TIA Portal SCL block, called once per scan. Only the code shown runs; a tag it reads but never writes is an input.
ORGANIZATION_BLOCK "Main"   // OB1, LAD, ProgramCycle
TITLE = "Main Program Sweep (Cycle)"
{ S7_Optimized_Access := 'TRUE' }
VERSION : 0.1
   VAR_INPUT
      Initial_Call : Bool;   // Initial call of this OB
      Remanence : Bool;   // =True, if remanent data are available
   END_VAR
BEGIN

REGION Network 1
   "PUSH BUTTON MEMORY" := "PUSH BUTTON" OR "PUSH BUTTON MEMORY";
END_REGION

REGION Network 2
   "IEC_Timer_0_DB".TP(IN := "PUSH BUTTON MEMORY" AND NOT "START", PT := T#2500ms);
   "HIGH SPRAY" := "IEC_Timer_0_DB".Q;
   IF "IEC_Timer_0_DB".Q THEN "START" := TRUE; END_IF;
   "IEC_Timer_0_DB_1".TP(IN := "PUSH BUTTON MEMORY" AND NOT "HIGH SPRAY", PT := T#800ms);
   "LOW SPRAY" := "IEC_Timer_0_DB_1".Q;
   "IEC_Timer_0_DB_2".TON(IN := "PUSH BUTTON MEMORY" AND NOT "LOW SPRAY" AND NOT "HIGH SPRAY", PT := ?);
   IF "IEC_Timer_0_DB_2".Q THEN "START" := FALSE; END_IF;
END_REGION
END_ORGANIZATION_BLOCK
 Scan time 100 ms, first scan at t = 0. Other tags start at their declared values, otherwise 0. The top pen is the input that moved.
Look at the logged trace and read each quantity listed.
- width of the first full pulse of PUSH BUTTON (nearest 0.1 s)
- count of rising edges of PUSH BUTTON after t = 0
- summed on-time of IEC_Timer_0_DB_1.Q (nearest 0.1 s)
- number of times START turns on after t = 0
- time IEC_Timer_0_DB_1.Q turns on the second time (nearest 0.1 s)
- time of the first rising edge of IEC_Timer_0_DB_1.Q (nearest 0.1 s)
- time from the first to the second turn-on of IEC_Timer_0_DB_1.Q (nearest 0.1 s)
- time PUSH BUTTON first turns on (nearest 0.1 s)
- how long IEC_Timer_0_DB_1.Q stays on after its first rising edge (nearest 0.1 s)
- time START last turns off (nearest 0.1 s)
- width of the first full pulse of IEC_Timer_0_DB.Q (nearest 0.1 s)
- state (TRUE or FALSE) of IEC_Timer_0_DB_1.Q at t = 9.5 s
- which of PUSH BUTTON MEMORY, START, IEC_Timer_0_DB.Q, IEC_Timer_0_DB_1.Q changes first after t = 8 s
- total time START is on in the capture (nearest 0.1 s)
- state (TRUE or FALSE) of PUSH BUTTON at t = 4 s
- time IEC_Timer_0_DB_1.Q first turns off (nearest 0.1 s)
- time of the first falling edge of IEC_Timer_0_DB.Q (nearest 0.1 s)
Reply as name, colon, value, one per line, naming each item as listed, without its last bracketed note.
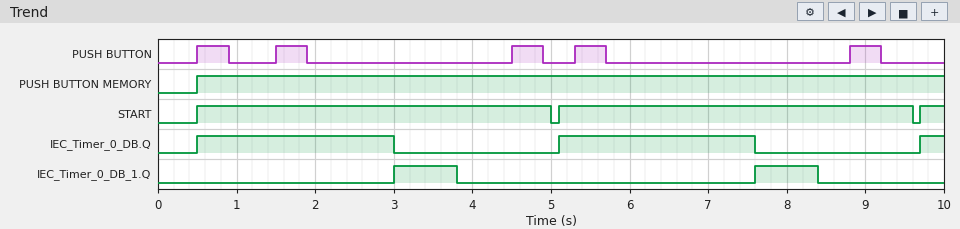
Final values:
width of the first full pulse of PUSH BUTTON: 0.4 s
count of rising edges of PUSH BUTTON after t = 0: 5
summed on-time of IEC_Timer_0_DB_1.Q: 1.6 s
number of times START turns on after t = 0: 3
time IEC_Timer_0_DB_1.Q turns on the second time: 7.6 s
time of the first rising edge of IEC_Timer_0_DB_1.Q: 3.0 s
time from the first to the second turn-on of IEC_Timer_0_DB_1.Q: 4.6 s
time PUSH BUTTON first turns on: 0.5 s
how long IEC_Timer_0_DB_1.Q stays on after its first rising edge: 0.8 s
time START last turns off: 9.6 s
width of the first full pulse of IEC_Timer_0_DB.Q: 2.5 s
state (TRUE or FALSE) of IEC_Timer_0_DB_1.Q at t = 9.5 s: FALSE
which of PUSH BUTTON MEMORY, START, IEC_Timer_0_DB.Q, IEC_Timer_0_DB_1.Q changes first after t = 8 s: IEC_Timer_0_DB_1.Q
total time START is on in the capture: 9.3 s
state (TRUE or FALSE) of PUSH BUTTON at t = 4 s: FALSE
time IEC_Timer_0_DB_1.Q first turns off: 3.8 s
time of the first falling edge of IEC_Timer_0_DB.Q: 3.0 s
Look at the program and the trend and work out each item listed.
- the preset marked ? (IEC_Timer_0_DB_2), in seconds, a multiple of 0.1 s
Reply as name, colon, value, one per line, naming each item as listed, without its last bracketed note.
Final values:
the preset marked ? (IEC_Timer_0_DB_2), in seconds, a multiple of 0.1 s: 1.2 s
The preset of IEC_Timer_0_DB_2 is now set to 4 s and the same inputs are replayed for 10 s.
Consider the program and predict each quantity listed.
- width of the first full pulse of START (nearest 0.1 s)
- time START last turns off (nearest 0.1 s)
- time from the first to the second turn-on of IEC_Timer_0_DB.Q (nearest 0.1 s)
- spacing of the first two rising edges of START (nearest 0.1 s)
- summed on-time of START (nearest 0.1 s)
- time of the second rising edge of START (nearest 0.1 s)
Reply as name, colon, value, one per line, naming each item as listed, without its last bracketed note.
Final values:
width of the first full pulse of START: 7.3 s
time START last turns off: 7.8 s
time from the first to the second turn-on of IEC_Timer_0_DB.Q: 7.4 s
spacing of the first two rising edges of START: 7.4 s
summed on-time of START: 9.4 s
time of the second rising edge of START: 7.9 s
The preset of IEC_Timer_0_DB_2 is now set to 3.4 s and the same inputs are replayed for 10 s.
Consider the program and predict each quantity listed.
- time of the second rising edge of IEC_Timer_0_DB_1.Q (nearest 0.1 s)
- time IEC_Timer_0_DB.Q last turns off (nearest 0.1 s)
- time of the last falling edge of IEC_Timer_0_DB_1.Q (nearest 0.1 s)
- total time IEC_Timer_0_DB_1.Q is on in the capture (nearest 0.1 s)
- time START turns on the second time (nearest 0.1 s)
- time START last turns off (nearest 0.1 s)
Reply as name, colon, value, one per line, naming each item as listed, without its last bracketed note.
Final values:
time of the second rising edge of IEC_Timer_0_DB_1.Q: 9.8 s
time IEC_Timer_0_DB.Q last turns off: 9.8 s
time of the last falling edge of IEC_Timer_0_DB_1.Q: 3.8 s
total time IEC_Timer_0_DB_1.Q is on in the capture: 1.0 s
time START turns on the second time: 7.3 s
time START last turns off: 7.2 s
